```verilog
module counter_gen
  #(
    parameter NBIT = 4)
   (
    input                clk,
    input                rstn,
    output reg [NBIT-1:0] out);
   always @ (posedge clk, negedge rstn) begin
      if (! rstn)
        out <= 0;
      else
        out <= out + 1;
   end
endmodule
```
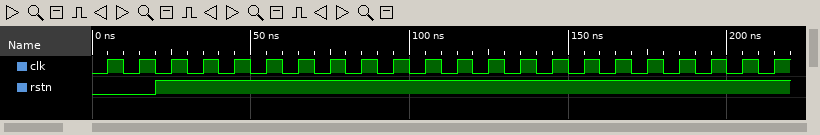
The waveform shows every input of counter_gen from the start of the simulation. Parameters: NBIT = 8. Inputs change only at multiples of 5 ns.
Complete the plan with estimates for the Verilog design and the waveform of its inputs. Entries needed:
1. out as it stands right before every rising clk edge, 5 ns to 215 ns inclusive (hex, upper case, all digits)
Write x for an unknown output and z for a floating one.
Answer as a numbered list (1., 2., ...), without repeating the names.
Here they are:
1. 00, 00, 00, 01, 02, 03, 04, 05, 06, 07, 08, 09, 0A, 0B, 0C, 0D, 0E, 0F, 10, 11, 12, 13
